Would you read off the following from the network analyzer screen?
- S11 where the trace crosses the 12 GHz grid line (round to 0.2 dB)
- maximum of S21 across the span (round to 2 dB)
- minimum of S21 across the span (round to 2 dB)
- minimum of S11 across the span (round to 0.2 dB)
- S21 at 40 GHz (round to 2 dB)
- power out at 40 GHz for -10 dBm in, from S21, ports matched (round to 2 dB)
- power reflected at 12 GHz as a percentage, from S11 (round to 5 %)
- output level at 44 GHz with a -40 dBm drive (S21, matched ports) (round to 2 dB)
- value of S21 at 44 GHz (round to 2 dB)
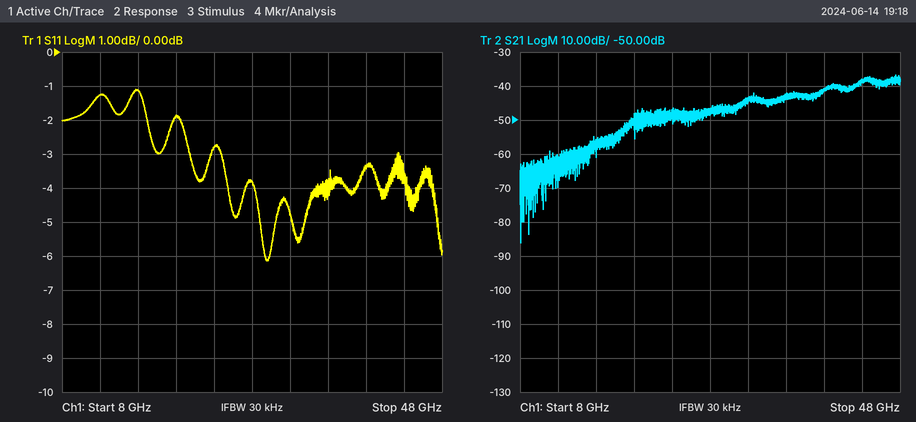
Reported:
-1.2 dB
-36 dB
-86 dB
-6.2 dB
-42 dB
-52 dBm
75 %
-78 dBm
-38 dB
